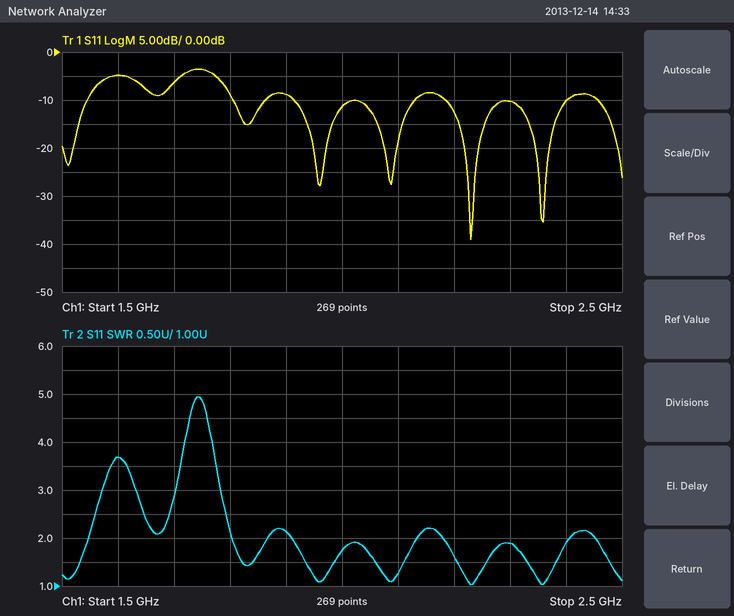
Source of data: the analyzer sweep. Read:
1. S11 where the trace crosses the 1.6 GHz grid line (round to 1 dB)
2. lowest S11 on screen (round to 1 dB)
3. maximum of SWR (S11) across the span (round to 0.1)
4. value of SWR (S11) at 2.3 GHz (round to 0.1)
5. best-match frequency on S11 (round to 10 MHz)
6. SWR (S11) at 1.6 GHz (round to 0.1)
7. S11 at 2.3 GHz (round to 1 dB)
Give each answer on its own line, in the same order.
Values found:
-5 dB
-39 dB
4.9
1.9
2.23 GHz
3.7
-10 dB
